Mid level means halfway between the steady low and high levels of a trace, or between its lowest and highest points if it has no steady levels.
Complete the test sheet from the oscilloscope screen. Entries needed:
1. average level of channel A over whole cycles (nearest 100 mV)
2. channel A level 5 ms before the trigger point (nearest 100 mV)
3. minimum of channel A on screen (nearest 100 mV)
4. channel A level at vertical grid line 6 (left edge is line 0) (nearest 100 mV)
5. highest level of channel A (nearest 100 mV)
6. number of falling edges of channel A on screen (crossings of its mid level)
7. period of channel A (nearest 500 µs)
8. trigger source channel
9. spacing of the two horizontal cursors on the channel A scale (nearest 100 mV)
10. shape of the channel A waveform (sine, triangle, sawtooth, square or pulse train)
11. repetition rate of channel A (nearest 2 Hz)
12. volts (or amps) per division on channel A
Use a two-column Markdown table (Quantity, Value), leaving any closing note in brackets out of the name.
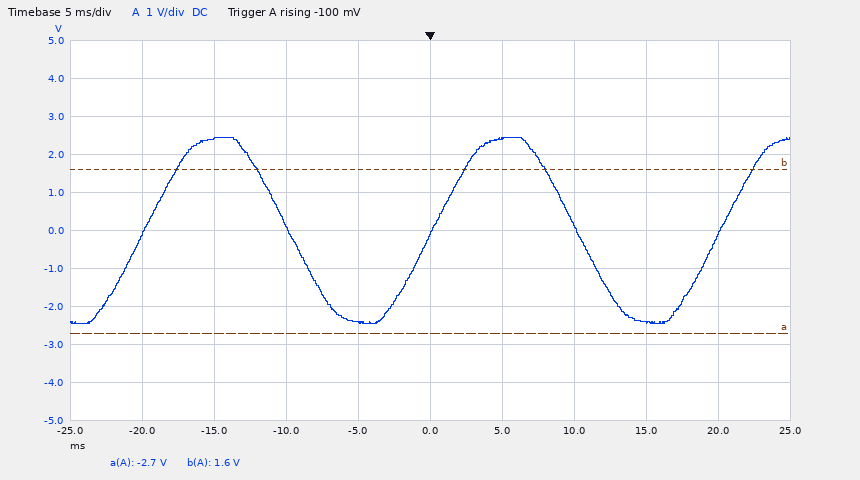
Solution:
| Quantity | Value |
|---|---|
| average level of channel A over whole cycles | 0.0 V |
| channel A level 5 ms before the trigger point | -2.4 V |
| minimum of channel A on screen | -2.4 V |
| channel A level at vertical grid line 6 (left edge is line 0) | 2.4 V |
| highest level of channel A | 2.4 V |
| number of falling edges of channel A on screen | 2 |
| period of channel A | 20.0 ms |
| trigger source channel | channel A |
| spacing of the two horizontal cursors on the channel A scale | 4.3 V |
| shape of the channel A waveform | sine |
| repetition rate of channel A | 50 Hz |
| volts (or amps) per division on channel A | 1 V |
